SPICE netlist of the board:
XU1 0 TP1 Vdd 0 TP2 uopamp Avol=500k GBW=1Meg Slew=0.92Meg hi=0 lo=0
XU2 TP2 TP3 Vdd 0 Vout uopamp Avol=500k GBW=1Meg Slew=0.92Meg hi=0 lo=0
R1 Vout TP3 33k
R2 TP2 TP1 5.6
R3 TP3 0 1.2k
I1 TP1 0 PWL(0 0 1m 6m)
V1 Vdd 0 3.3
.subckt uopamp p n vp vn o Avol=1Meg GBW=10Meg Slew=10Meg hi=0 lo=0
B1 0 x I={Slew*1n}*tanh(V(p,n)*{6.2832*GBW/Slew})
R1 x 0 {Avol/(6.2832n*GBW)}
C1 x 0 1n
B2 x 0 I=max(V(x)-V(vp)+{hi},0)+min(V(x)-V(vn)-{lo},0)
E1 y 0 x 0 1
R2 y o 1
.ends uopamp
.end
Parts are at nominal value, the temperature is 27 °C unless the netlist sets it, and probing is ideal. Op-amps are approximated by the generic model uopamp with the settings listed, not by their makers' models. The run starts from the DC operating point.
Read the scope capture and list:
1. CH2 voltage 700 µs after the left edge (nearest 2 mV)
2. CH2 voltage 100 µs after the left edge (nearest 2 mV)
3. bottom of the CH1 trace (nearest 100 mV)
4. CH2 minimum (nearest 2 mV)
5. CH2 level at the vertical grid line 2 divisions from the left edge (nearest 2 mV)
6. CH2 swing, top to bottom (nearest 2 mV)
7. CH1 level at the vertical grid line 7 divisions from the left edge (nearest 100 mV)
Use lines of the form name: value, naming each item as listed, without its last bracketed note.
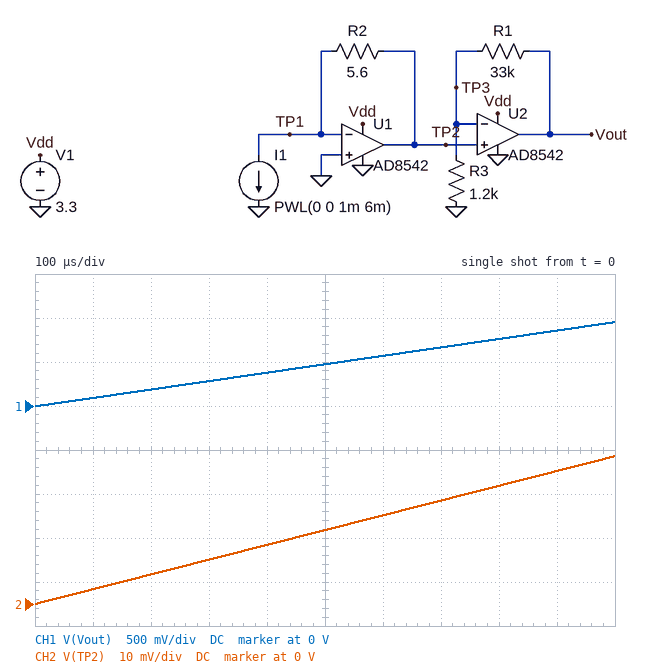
CH2 voltage 700 µs after the left edge: 24 mV
CH2 voltage 100 µs after the left edge: 4 mV
bottom of the CH1 trace: 0 V
CH2 minimum: 0 V
CH2 level at the vertical grid line 2 divisions from the left edge: 6 mV
CH2 swing, top to bottom: 34 mV
CH1 level at the vertical grid line 7 divisions from the left edge: 700 mV
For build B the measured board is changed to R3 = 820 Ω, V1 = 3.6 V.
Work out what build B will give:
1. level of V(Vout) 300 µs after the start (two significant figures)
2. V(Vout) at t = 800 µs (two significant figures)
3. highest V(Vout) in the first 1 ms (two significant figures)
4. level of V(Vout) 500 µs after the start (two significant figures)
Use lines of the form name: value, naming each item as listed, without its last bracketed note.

level of V(Vout) 300 µs after the start: 410 mV
V(Vout) at t = 800 µs: 1.1 V
highest V(Vout) in the first 1 ms: 1.4 V
level of V(Vout) 500 µs after the start: 680 mV
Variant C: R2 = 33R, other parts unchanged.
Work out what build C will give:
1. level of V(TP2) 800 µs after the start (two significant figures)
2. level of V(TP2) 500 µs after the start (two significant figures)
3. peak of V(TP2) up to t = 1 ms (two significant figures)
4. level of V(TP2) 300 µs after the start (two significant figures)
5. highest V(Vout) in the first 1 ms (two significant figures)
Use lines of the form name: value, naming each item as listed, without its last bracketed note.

level of V(TP2) 800 µs after the start: 160 mV
level of V(TP2) 500 µs after the start: 99 mV
peak of V(TP2) up to t = 1 ms: 200 mV
level of V(TP2) 300 µs after the start: 59 mV
highest V(Vout) in the first 1 ms: 3.3 V
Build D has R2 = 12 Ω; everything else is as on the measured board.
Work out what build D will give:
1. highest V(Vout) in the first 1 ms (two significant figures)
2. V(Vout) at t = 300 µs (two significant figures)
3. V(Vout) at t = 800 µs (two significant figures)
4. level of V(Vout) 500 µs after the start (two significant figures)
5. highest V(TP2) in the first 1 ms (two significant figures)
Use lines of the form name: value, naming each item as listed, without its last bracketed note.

highest V(Vout) in the first 1 ms: 2.0 V
V(Vout) at t = 300 µs: 610 mV
V(Vout) at t = 800 µs: 1.6 V
level of V(Vout) 500 µs after the start: 1.0 V
highest V(TP2) in the first 1 ms: 72 mV
